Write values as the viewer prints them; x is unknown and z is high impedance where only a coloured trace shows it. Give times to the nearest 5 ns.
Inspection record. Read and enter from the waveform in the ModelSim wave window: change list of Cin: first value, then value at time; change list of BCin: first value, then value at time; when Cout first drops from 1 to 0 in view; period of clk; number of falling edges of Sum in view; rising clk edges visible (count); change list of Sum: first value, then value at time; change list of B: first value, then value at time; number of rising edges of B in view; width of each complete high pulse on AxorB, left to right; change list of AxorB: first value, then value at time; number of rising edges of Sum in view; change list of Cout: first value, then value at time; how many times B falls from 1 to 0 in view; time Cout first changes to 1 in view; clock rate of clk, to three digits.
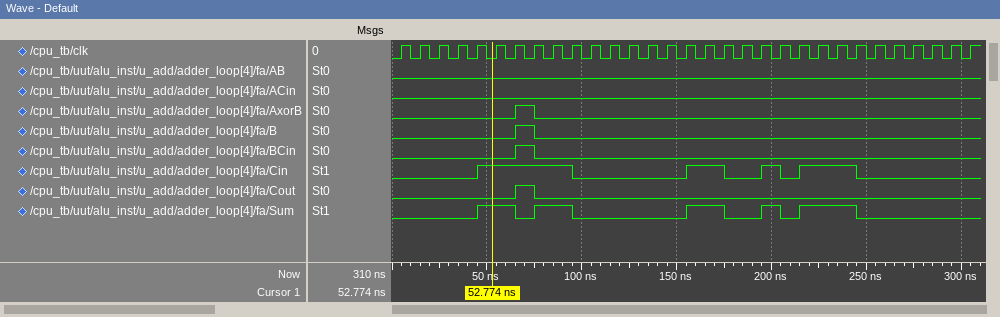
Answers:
0, 1 at 45 ns, 0 at 95 ns, 1 at 155 ns, 0 at 175 ns, 1 at 195 ns, 0 at 205 ns, 1 at 215 ns, 0 at 245 ns
0, 1 at 65 ns, 0 at 75 ns
75 ns
10 ns
5
31
0, 1 at 45 ns, 0 at 65 ns, 1 at 75 ns, 0 at 95 ns, 1 at 155 ns, 0 at 175 ns, 1 at 195 ns, 0 at 205 ns, 1 at 215 ns, 0 at 245 ns
0, 1 at 65 ns, 0 at 75 ns
1
10 ns
0, 1 at 65 ns, 0 at 75 ns
5
0, 1 at 65 ns, 0 at 75 ns
1
65 ns
100 MHz
